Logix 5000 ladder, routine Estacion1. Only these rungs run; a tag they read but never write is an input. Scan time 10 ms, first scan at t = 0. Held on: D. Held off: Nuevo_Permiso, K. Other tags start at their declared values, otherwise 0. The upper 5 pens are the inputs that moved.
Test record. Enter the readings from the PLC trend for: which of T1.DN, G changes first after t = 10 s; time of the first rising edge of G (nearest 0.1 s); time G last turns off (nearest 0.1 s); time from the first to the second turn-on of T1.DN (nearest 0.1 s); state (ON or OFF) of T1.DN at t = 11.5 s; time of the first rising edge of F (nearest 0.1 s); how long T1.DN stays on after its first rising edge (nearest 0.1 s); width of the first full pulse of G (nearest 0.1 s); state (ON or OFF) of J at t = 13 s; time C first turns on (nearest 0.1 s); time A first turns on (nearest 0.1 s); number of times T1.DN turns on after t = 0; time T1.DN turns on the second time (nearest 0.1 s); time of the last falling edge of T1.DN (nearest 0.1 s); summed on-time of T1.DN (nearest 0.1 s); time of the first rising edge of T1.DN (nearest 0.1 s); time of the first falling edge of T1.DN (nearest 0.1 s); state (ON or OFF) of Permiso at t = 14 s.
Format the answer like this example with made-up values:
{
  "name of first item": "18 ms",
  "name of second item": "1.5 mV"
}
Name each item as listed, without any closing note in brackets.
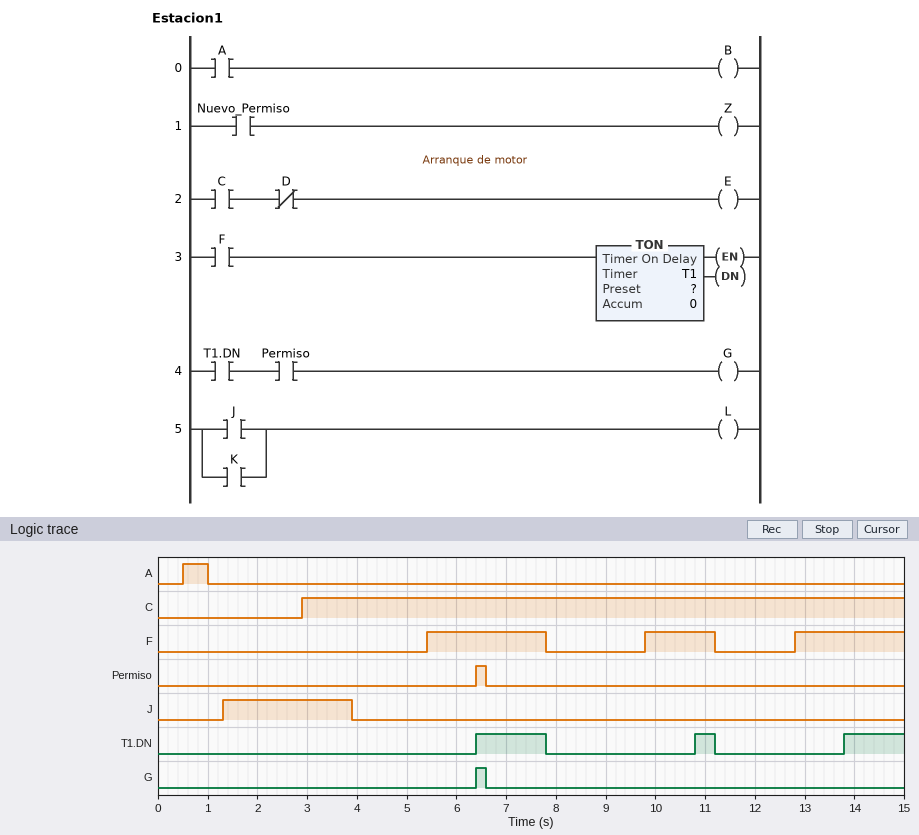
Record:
{
  "which of T1.DN, G changes first after t = 10 s": "T1.DN",
  "time of the first rising edge of G": "6.4 s",
  "time G last turns off": "6.6 s",
  "time from the first to the second turn-on of T1.DN": "4.4 s",
  "state (ON or OFF) of T1.DN at t = 11.5 s": "OFF",
  "time of the first rising edge of F": "5.4 s",
  "how long T1.DN stays on after its first rising edge": "1.4 s",
  "width of the first full pulse of G": "0.2 s",
  "state (ON or OFF) of J at t = 13 s": "OFF",
  "time C first turns on": "2.9 s",
  "time A first turns on": "0.5 s",
  "number of times T1.DN turns on after t = 0": "3",
  "time T1.DN turns on the second time": "10.8 s",
  "time of the last falling edge of T1.DN": "11.2 s",
  "summed on-time of T1.DN": "3.0 s",
  "time of the first rising edge of T1.DN": "6.4 s",
  "time of the first falling edge of T1.DN": "7.8 s",
  "state (ON or OFF) of Permiso at t = 14 s": "OFF"
}
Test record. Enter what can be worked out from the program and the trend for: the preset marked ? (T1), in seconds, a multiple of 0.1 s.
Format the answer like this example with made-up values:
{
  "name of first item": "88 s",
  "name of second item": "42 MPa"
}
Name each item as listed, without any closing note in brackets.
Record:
{
  "the preset marked ? (T1), in seconds, a multiple of 0.1 s": "1.0 s"
}
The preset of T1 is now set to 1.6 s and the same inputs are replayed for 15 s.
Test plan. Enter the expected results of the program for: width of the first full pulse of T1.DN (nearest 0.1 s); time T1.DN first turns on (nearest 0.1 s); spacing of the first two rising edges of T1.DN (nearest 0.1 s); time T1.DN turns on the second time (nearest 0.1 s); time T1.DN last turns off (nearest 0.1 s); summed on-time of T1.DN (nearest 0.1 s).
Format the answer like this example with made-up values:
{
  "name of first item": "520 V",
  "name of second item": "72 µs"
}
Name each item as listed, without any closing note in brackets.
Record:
{
  "width of the first full pulse of T1.DN": "0.8 s",
  "time T1.DN first turns on": "7.0 s",
  "spacing of the first two rising edges of T1.DN": "7.4 s",
  "time T1.DN turns on the second time": "14.4 s",
  "time T1.DN last turns off": "7.8 s",
  "summed on-time of T1.DN": "1.4 s"
}
